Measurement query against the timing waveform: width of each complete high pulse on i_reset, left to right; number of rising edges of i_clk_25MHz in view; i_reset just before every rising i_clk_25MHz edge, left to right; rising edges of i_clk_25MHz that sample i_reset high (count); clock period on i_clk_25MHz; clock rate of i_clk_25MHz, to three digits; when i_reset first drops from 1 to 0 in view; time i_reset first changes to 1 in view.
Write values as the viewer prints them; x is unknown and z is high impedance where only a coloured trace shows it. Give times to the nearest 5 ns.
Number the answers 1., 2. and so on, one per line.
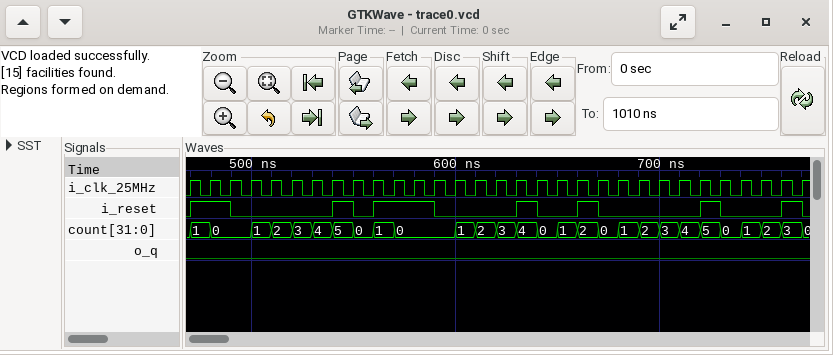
1. 20 ns, 10 ns, 30 ns, 10 ns, 10 ns, 10 ns, 10 ns
2. 31
3. 0 1 1 0 0 0 0 0 1 0 1 1 1 0 0 0 0 1 0 0 1 0 0 0 0 0 1 0 0 0 1
4. 10
5. 10 ns
6. 100 MHz
7. 490 ns
8. 470 ns
